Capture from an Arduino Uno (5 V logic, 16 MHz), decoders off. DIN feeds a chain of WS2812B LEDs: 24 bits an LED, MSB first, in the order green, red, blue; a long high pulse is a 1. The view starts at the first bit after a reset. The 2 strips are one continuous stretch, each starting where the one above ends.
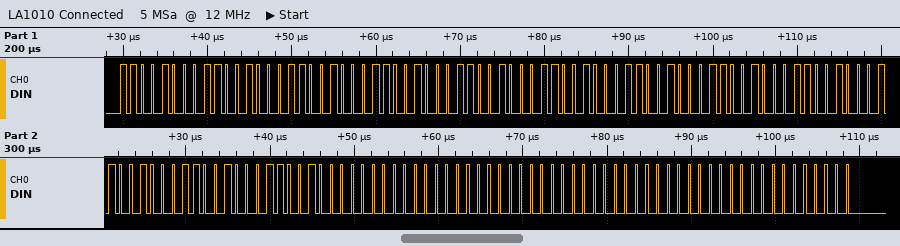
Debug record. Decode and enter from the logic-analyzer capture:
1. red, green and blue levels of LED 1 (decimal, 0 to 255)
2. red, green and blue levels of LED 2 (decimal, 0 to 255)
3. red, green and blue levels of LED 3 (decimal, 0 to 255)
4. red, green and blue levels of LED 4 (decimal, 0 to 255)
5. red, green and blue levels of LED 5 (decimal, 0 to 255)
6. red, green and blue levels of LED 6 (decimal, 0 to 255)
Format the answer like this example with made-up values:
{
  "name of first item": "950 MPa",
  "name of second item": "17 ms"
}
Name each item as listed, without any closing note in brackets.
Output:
{
  "red, green and blue levels of LED 1": "200, 200, 200",
  "red, green and blue levels of LED 2": "200, 200, 200",
  "red, green and blue levels of LED 3": "200, 200, 200",
  "red, green and blue levels of LED 4": "200, 200, 200",
  "red, green and blue levels of LED 5": "0, 0, 0",
  "red, green and blue levels of LED 6": "0, 0, 0"
}
